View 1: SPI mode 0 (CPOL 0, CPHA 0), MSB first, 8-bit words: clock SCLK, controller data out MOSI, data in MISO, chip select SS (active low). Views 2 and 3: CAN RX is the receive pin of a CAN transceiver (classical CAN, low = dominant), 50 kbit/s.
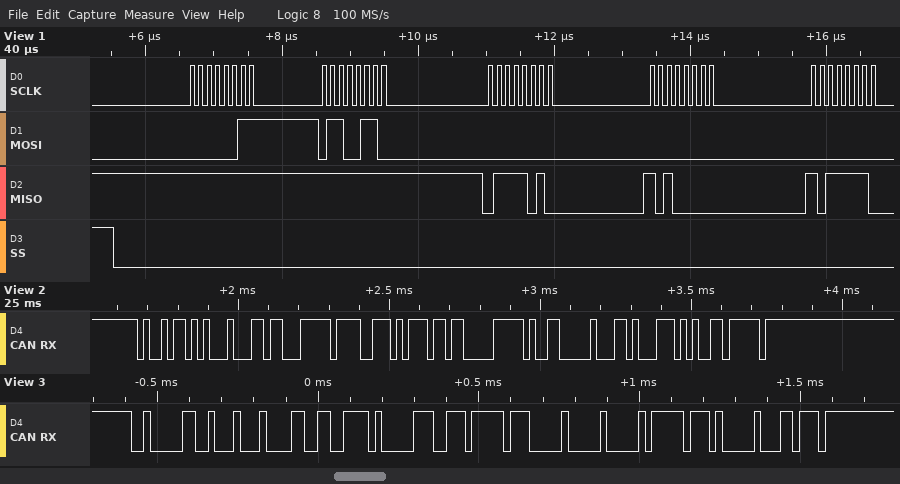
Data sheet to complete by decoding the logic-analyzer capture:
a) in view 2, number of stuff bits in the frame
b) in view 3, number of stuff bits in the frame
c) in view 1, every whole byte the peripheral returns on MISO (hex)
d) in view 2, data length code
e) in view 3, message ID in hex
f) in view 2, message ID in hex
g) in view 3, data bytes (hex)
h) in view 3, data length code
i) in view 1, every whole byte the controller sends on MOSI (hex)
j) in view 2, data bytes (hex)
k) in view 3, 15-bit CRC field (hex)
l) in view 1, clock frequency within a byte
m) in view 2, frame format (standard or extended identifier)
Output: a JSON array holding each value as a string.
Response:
["4", "8", "0xFF 0xFF 0x7A 0xA0 0xBE", "8", "0x209", "0x4B5", "86 67 A0 CE FF 00 00 FF", "8", "0x03 0x66 0x00 0x00 0x00", "D8 FF 9D 76 C1 F3 00 D1", "0x201B", "8 MHz", "standard"]
